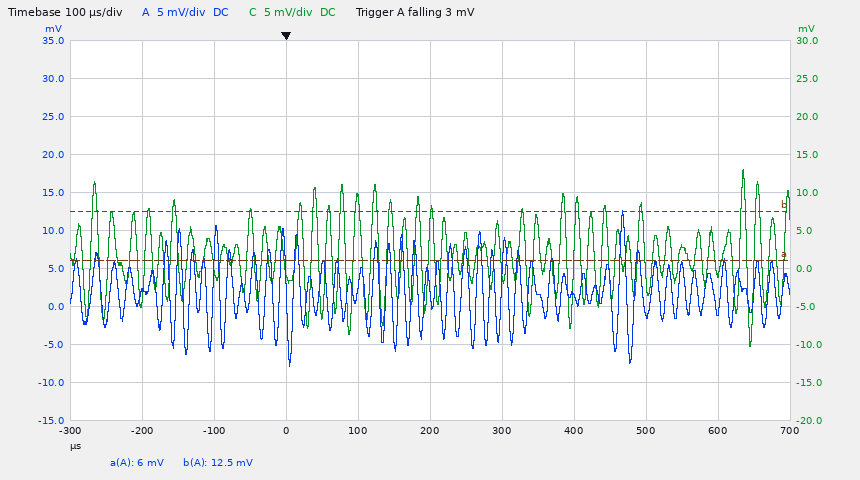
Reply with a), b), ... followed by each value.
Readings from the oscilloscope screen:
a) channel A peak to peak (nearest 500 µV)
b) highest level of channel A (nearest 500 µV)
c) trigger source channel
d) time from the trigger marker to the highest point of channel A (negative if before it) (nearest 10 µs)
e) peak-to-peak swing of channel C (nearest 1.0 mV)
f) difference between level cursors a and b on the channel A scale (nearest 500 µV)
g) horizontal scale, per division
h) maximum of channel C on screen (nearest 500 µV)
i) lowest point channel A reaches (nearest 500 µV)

a) 20.5 mV
b) 12.5 mV
c) channel A
d) +470 µs
e) 23.0 mV
f) 6.5 mV
g) 100 µs
h) 13.0 mV
i) -8.0 mV
